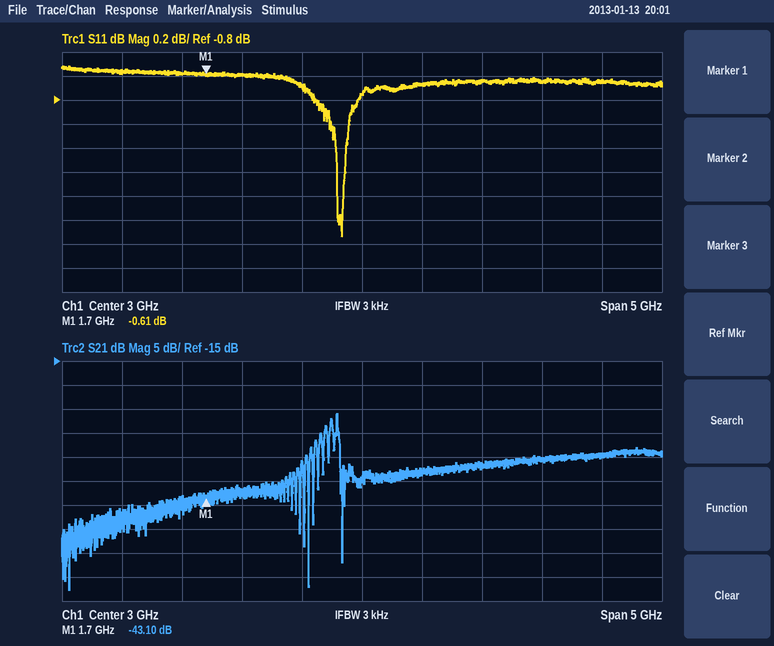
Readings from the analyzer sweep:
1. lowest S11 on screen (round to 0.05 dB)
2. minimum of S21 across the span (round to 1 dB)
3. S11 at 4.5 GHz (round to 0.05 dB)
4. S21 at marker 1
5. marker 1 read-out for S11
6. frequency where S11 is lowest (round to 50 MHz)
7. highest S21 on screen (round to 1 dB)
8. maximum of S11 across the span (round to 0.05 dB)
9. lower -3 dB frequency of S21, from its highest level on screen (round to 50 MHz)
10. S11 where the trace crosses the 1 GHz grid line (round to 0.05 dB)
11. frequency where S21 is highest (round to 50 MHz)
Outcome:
-1.95 dB
-63 dB
-0.65 dB
-43.10 dB
-0.61 dB
2.85 GHz
-26 dB
-0.50 dB
2.80 GHz
-0.55 dB
2.80 GHz
